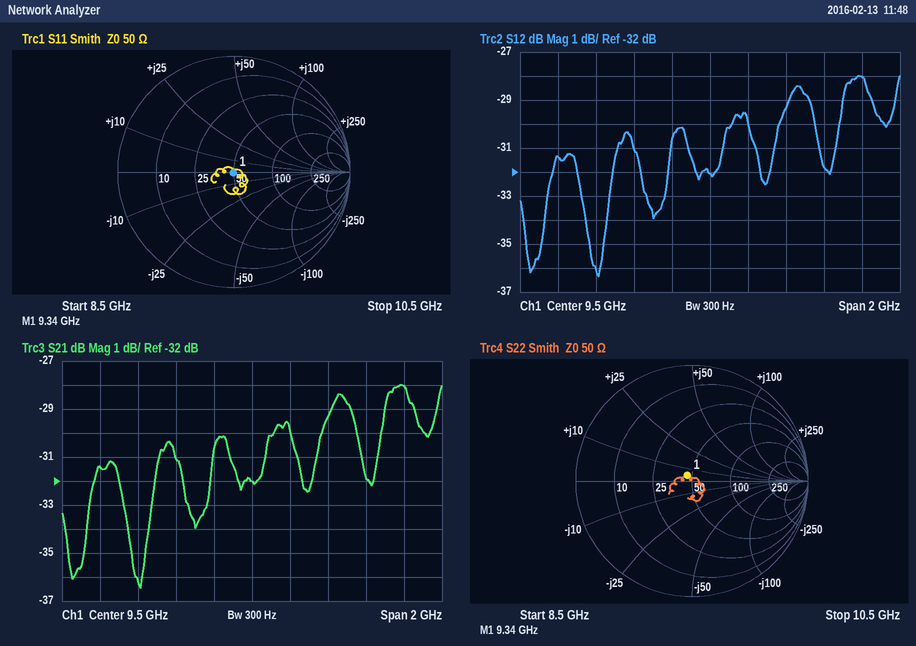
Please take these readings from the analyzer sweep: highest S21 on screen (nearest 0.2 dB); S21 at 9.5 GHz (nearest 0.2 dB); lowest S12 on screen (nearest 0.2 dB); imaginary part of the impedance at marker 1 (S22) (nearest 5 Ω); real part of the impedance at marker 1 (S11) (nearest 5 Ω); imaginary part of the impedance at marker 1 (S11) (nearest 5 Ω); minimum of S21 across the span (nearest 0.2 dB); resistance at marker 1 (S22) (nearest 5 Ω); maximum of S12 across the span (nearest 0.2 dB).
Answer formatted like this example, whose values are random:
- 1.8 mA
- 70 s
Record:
- -28.0 dB
- -32.0 dB
- -36.4 dB
- +5 Ω
- 50 Ω
- 0 Ω
- -36.4 dB
- 45 Ω
- -28.0 dB
